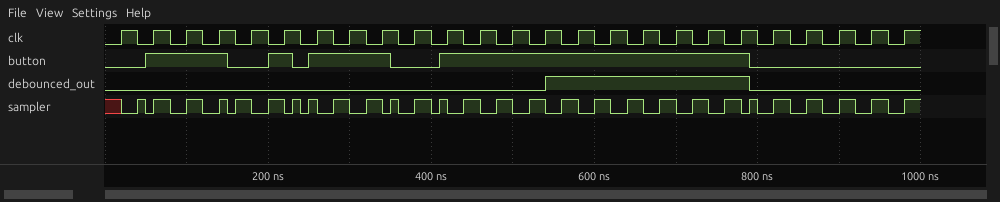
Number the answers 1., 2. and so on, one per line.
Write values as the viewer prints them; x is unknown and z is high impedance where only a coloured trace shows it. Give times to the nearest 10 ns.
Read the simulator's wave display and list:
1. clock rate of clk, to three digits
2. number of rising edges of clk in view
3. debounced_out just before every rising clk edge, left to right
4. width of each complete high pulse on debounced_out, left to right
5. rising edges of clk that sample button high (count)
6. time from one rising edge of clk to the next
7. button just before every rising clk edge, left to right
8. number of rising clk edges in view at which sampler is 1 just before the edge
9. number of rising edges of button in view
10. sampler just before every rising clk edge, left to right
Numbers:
1. 25.0 MHz
2. 25
3. 0 0 0 0 0 0 0 0 0 0 0 0 0 0 1 1 1 1 1 1 0 0 0 0 0
4. 250 ns
5. 17
6. 40 ns
7. 0 1 1 1 0 1 1 1 1 0 1 1 1 1 1 1 1 1 1 1 0 0 0 0 0
8. 15
9. 4
10. x 0 0 0 1 1 1 1 1 0 1 1 1 1 1 1 1 1 1 1 0 0 0 0 0
